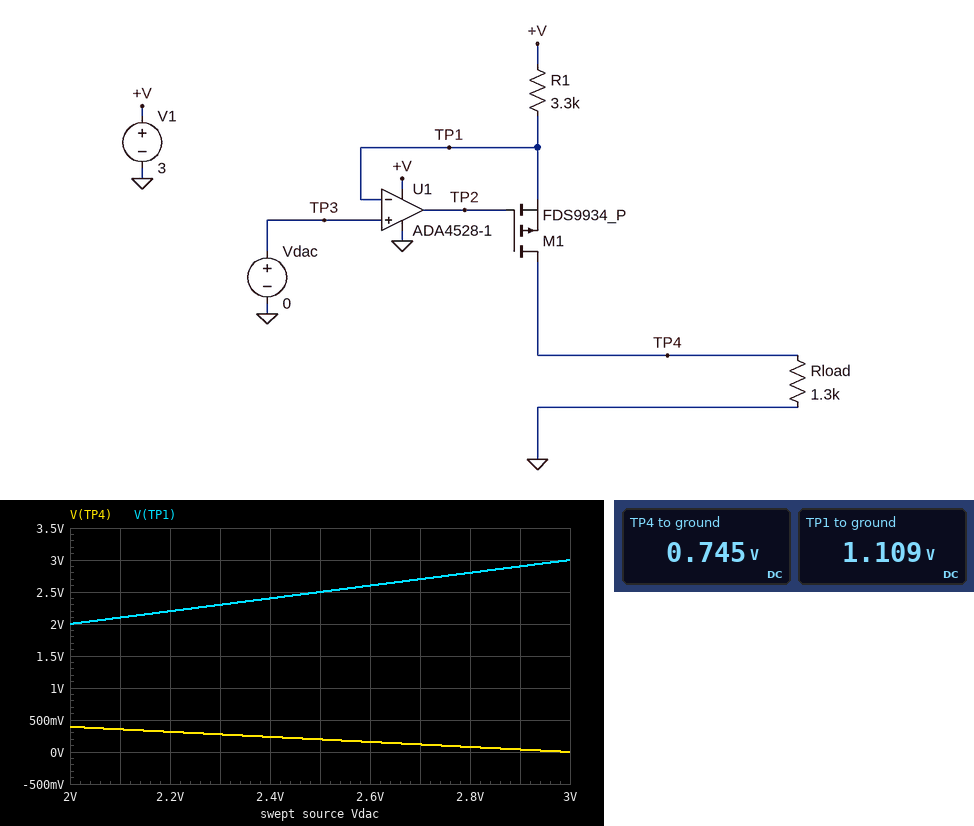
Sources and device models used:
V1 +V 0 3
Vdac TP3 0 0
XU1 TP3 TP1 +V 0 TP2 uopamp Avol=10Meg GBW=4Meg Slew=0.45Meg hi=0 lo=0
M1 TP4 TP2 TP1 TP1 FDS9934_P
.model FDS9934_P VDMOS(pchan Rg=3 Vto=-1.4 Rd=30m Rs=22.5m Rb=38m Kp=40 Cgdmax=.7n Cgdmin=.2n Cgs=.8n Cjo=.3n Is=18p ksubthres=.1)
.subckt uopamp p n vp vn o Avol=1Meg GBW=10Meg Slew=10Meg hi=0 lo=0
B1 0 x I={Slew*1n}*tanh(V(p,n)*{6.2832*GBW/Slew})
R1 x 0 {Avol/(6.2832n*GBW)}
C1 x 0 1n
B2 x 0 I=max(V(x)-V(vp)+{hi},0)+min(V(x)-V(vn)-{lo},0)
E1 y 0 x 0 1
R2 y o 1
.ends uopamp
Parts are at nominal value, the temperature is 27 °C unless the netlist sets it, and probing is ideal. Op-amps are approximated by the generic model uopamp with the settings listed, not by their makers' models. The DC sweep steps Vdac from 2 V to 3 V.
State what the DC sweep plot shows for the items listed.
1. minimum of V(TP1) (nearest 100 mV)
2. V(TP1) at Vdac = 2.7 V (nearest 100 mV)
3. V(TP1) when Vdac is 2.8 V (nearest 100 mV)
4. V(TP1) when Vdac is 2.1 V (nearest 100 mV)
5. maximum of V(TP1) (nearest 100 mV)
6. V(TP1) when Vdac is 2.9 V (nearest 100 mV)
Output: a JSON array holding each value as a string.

["2.0 V", "2.7 V", "2.8 V", "2.1 V", "3.0 V", "2.9 V"]
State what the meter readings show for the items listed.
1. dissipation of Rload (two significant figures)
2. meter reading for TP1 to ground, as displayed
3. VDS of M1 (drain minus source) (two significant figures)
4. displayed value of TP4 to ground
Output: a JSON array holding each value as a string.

["430 µW", "1.109 V", "-360 mV", "0.745 V"]
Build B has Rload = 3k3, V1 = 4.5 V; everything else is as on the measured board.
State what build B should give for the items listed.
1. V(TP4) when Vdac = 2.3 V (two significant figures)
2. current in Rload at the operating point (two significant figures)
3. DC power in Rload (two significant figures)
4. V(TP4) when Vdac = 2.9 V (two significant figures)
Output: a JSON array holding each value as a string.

["2.2 V", "680 µA", "1.5 mW", "1.6 V"]
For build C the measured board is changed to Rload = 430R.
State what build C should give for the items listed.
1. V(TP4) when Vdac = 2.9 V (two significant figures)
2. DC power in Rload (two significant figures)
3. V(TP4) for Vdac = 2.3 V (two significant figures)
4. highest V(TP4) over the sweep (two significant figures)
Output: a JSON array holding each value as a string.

["13 mV", "140 µW", "91 mV", "130 mV"]
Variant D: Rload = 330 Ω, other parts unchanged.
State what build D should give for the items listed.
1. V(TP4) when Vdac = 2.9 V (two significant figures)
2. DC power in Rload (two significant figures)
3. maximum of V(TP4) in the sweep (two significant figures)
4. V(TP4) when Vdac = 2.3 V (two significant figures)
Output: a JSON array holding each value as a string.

["10 mV", "110 µW", "100 mV", "70 mV"]
